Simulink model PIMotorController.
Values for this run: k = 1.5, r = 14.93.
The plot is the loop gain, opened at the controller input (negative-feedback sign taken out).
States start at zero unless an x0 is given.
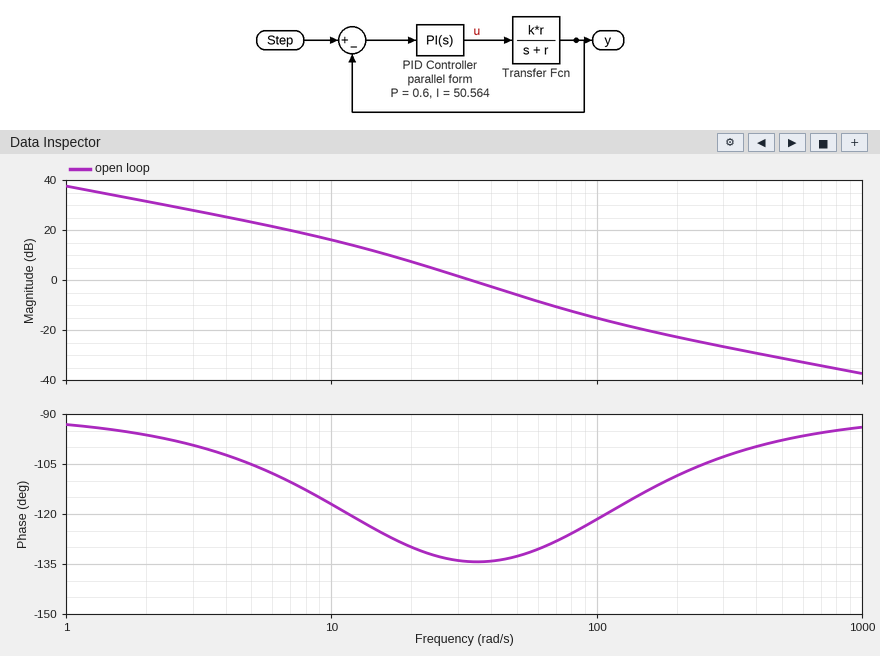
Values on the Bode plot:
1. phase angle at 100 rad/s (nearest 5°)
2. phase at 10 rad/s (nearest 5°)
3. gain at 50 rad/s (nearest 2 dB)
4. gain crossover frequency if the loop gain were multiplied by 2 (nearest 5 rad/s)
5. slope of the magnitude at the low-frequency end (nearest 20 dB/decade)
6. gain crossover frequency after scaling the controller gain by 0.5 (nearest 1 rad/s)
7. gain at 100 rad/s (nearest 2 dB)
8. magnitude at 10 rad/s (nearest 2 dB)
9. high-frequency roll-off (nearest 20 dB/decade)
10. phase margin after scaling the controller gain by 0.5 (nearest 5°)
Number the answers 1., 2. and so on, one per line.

1. -120°
2. -115°
3. -6 dB
4. 50 rad/s
5. -20 dB/decade
6. 22 rad/s
7. -16 dB
8. 16 dB
9. -20 dB/decade
10. 50°
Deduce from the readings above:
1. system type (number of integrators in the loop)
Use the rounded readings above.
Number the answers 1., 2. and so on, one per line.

1. 1
